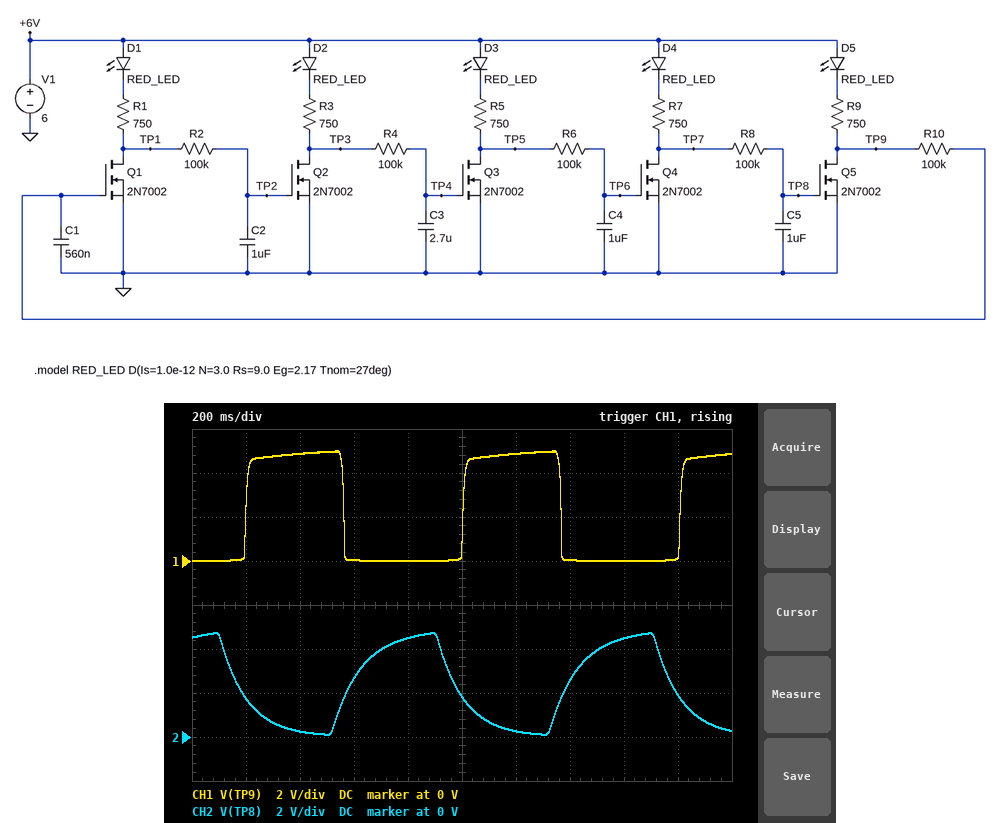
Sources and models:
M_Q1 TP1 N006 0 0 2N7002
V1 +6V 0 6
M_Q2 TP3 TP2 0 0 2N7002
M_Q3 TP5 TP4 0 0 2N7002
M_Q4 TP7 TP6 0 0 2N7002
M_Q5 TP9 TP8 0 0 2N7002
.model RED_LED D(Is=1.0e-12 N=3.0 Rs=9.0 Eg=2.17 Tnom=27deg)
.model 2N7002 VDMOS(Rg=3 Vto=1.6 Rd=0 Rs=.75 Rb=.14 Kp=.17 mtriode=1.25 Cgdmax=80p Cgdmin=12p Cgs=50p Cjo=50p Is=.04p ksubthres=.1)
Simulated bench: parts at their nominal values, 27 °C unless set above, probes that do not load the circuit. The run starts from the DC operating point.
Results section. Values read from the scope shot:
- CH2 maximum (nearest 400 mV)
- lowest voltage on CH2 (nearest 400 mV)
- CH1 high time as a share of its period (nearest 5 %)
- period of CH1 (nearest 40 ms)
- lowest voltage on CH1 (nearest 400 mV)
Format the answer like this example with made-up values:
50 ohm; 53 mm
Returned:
4.8 V; 0 V; 45 %; 800 ms; 0 V
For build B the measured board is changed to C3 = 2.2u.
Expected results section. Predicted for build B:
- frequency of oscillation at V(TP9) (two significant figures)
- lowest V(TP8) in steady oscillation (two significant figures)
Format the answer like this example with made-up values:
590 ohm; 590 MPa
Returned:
1.3 Hz; 120 mV
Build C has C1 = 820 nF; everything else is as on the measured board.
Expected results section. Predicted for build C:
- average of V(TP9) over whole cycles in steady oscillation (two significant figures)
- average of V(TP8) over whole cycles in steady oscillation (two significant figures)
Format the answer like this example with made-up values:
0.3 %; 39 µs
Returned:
2.1 V; 2.4 V
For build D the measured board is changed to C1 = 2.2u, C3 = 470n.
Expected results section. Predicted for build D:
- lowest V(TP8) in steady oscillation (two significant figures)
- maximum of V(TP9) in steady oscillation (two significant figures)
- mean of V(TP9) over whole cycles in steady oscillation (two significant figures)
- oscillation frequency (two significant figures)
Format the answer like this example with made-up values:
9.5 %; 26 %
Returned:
130 mV; 4.7 V; 2.1 V; 1.3 Hz
